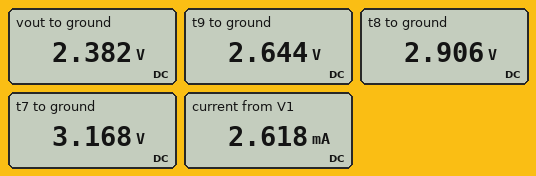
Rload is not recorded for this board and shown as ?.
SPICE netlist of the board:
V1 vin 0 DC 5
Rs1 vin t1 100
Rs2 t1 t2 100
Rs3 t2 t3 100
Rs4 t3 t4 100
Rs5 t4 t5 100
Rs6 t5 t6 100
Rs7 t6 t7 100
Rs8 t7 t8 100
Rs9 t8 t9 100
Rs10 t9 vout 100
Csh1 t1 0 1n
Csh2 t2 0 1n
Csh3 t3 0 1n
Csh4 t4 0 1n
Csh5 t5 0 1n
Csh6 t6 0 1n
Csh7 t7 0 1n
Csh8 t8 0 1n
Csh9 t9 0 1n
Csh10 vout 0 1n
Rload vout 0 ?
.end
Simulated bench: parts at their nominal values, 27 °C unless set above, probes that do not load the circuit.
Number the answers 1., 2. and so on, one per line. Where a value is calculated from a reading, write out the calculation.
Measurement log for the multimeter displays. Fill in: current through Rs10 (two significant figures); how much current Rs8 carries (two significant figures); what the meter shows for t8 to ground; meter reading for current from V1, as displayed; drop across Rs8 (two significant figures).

1. (2.644 V - 2.382 V) / 100 Ω = 2.6 mA
2. (3.168 V - 2.906 V) / 100 Ω = 2.6 mA
3. 2.906 V
4. 2.618 mA
5. 3.168 V - 2.906 V = 260 mV
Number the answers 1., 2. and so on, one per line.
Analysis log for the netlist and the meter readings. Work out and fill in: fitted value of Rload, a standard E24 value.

1. 910 Ω
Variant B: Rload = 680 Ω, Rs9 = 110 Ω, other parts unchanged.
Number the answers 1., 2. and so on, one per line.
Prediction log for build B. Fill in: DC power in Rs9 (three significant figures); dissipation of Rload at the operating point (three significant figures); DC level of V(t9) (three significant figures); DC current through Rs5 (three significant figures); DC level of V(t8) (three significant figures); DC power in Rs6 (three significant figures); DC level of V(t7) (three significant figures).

1. 963 µW
2. 5.95 mW
3. 2.31 V
4. 2.96 mA
5. 2.63 V
6. 875 µW
7. 2.93 V
